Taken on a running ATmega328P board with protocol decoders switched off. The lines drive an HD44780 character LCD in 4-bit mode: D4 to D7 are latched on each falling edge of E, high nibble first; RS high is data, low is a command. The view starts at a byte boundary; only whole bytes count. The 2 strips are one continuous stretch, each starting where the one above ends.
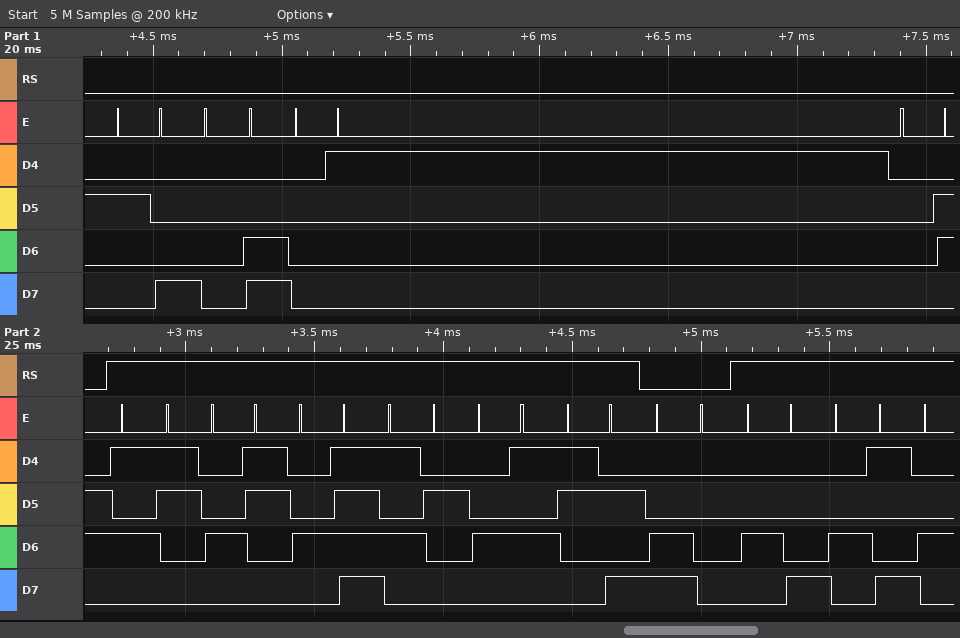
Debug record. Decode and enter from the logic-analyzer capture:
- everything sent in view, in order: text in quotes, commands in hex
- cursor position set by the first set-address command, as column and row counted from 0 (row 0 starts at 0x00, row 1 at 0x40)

0x28 0x0C 0x01 0x06 "SCORE:" 0xC0 "HI"
column 0, row 1
